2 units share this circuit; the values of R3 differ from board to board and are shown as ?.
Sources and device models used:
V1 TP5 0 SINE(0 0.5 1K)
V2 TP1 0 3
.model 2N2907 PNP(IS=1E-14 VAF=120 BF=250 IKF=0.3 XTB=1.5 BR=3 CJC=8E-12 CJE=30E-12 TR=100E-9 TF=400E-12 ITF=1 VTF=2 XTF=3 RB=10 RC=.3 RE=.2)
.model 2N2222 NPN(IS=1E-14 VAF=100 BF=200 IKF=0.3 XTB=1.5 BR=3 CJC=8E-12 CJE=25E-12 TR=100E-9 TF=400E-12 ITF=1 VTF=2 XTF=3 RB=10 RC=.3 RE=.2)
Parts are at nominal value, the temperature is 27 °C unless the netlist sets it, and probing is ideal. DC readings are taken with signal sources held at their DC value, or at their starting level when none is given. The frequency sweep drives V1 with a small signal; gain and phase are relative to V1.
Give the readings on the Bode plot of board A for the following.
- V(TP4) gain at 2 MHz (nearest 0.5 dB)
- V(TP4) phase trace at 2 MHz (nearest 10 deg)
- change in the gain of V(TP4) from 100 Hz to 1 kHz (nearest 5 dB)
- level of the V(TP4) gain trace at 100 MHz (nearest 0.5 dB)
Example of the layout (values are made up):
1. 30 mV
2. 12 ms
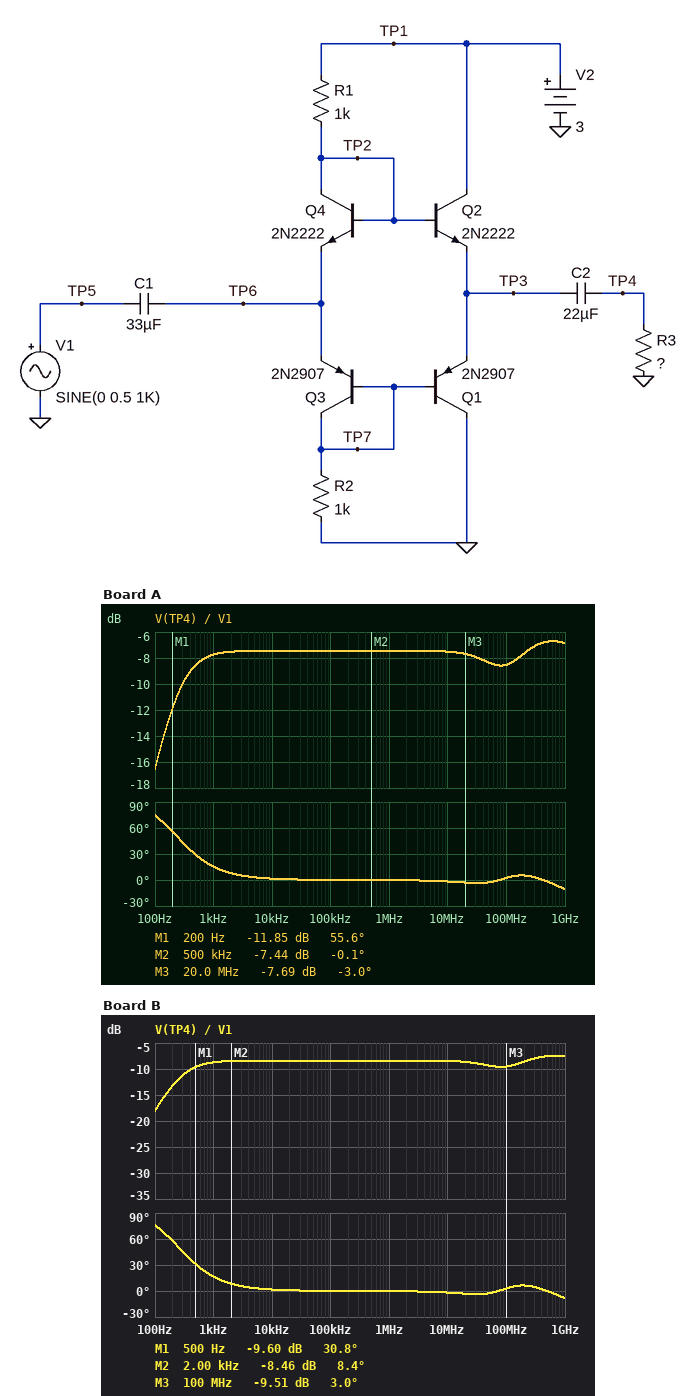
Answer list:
1. -7.5 dB
2. 0 deg
3. 10 dB
4. -8.5 dB
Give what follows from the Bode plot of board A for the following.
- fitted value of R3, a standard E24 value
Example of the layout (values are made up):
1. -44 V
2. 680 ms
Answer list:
1. 12 Ω
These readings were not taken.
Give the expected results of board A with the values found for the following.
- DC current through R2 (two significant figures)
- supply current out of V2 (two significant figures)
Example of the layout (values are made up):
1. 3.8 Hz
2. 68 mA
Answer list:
1. 850 µA
2. 1.7 mA
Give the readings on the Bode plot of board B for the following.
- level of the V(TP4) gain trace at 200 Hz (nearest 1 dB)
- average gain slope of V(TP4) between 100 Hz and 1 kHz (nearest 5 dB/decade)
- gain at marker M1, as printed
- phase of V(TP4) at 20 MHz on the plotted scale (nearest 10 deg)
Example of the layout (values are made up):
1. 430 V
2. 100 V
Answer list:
1. -13 dB
2. 10 dB/decade
3. -9.60 dB
4. 0 deg
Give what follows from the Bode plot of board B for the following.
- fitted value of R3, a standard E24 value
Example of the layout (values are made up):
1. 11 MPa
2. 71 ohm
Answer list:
1. 10 Ω
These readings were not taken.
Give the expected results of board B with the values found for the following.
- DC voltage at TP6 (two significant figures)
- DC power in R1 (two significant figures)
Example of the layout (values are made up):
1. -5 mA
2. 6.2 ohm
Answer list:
1. 1.5 V
2. 720 µW
